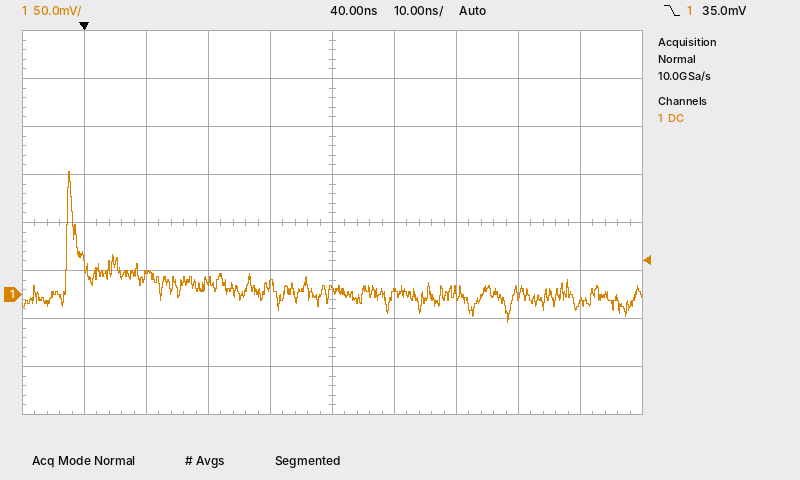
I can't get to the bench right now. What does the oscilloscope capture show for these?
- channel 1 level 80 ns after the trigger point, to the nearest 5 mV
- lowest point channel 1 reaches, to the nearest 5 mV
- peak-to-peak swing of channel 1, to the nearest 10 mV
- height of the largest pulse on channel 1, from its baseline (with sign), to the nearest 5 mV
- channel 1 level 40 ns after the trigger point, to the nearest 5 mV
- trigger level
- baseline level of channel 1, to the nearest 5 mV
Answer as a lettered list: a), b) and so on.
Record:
a) -10 mV
b) -30 mV
c) 160 mV
d) +125 mV
e) 5 mV
f) 35.0 mV
g) 0 mV
